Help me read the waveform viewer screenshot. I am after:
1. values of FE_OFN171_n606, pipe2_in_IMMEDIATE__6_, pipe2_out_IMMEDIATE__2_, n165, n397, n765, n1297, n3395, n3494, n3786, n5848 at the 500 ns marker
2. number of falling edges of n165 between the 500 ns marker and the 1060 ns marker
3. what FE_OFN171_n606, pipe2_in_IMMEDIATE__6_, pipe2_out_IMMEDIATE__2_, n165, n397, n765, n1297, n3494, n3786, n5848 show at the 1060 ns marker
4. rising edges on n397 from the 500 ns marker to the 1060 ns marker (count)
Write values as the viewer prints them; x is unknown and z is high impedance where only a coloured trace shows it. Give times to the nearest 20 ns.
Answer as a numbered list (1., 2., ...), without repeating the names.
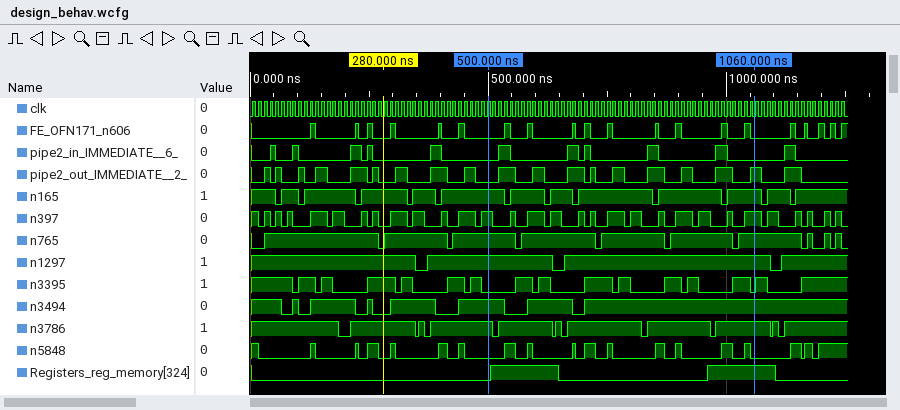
1. FE_OFN171_n606=0, pipe2_in_IMMEDIATE__6_=0, pipe2_out_IMMEDIATE__2_=0, n165=1, n397=1, n765=1, n1297=1, n3395=0, n3494=1, n3786=1, n5848=0
2. 5
3. FE_OFN171_n606=0, pipe2_in_IMMEDIATE__6_=0, pipe2_out_IMMEDIATE__2_=1, n165=1, n397=1, n765=1, n1297=1, n3494=1, n3786=1, n5848=0
4. 12
